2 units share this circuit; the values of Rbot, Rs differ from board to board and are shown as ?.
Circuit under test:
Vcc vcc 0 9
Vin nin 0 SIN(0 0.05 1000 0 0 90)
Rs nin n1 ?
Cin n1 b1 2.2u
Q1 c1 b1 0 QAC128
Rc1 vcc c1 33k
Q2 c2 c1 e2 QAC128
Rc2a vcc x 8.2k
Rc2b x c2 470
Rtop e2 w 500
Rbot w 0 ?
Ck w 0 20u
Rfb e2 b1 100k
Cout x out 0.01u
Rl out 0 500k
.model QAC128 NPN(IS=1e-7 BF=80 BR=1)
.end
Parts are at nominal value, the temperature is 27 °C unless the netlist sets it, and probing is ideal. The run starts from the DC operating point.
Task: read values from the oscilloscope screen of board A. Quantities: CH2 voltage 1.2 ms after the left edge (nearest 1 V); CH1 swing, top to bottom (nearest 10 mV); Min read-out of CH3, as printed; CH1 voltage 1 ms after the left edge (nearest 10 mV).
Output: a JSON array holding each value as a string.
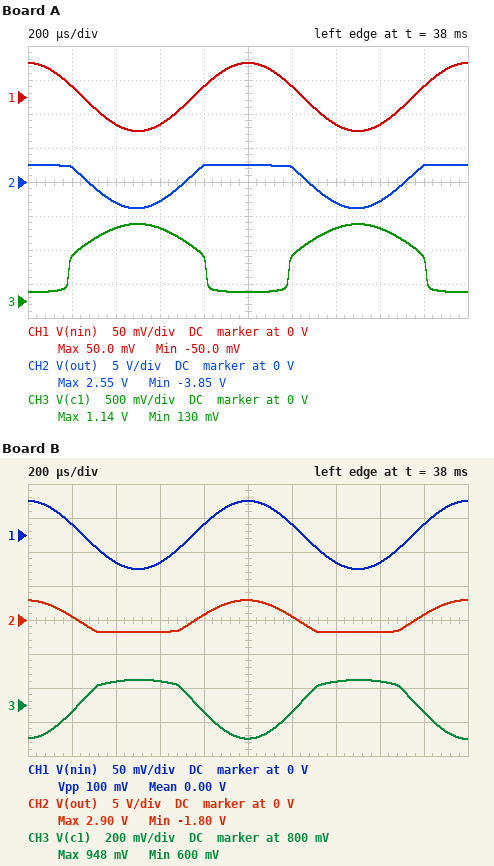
["2 V", "100 mV", "130 mV", "50 mV"]
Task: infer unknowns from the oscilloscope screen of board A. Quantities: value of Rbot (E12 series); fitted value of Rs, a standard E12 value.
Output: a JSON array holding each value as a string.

["1.5 kΩ", "15 kΩ"]
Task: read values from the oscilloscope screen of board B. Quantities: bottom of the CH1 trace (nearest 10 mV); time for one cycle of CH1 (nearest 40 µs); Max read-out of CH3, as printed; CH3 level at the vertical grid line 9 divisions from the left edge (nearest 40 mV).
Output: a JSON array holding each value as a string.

["-50 mV", "1.00 ms", "948 mV", "760 mV"]
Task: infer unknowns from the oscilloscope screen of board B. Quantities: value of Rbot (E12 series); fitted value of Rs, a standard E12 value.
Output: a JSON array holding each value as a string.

["270 Ω", "22 kΩ"]
